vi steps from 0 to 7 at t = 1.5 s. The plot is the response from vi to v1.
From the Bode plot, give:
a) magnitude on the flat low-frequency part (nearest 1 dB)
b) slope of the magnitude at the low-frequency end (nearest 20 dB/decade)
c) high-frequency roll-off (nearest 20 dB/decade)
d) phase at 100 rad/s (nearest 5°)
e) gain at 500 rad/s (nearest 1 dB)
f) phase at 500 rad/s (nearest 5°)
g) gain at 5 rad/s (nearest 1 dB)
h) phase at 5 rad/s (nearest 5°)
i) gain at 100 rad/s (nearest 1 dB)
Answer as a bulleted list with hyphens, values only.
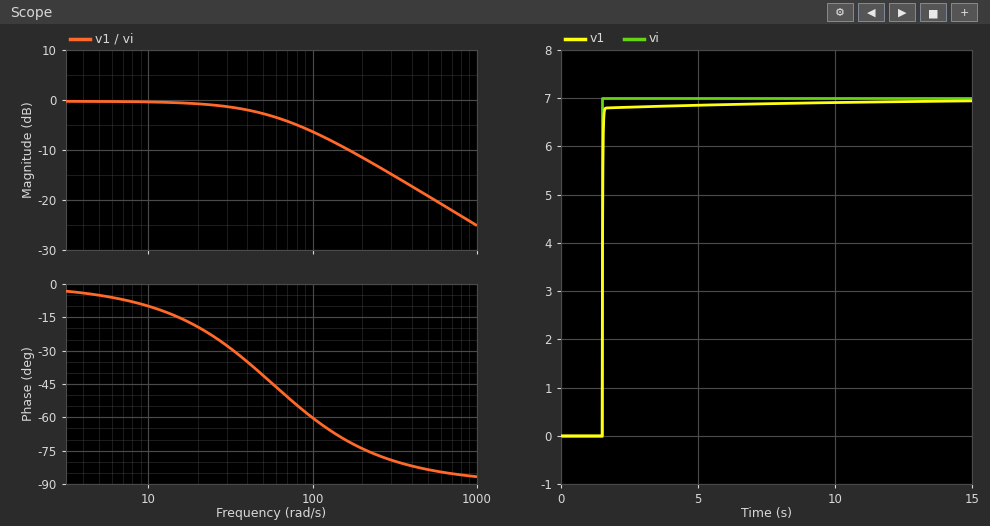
- 0 dB
- 0 dB/decade
- -20 dB/decade
- -60°
- -19 dB
- -85°
- 0 dB
- -5°
- -6 dB
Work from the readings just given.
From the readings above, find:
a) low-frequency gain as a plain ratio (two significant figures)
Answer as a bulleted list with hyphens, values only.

- 1.0
